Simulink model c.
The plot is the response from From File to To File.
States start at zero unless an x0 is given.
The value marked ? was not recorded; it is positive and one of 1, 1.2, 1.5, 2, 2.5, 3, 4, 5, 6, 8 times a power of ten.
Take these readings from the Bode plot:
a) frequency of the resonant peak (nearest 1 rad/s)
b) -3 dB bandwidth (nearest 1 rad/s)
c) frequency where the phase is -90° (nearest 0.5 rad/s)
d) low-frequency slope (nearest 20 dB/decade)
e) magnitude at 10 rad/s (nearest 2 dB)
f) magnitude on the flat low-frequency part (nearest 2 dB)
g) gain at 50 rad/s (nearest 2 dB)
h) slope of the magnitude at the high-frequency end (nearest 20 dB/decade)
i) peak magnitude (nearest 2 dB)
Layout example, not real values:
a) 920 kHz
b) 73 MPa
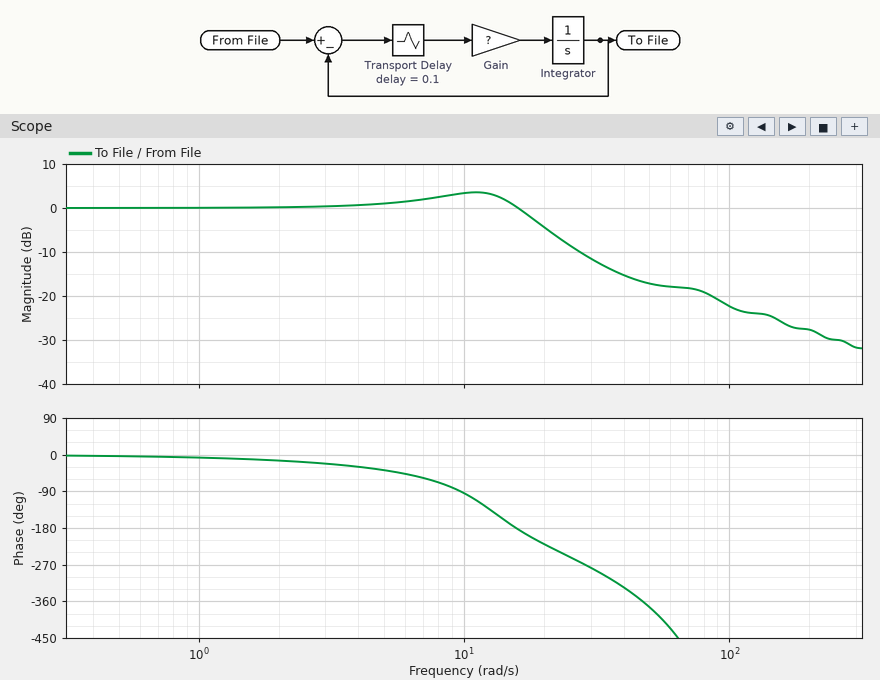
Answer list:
a) 11 rad/s
b) 19 rad/s
c) 9.5 rad/s
d) 0 dB/decade
e) 4 dB
f) 0 dB
g) -18 dB
h) -20 dB/decade
i) 4 dB
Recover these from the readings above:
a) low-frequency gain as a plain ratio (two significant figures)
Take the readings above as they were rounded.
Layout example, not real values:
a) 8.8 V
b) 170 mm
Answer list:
a) 1.0
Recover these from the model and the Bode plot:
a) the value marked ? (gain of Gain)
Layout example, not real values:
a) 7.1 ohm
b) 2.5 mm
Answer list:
a) 8
